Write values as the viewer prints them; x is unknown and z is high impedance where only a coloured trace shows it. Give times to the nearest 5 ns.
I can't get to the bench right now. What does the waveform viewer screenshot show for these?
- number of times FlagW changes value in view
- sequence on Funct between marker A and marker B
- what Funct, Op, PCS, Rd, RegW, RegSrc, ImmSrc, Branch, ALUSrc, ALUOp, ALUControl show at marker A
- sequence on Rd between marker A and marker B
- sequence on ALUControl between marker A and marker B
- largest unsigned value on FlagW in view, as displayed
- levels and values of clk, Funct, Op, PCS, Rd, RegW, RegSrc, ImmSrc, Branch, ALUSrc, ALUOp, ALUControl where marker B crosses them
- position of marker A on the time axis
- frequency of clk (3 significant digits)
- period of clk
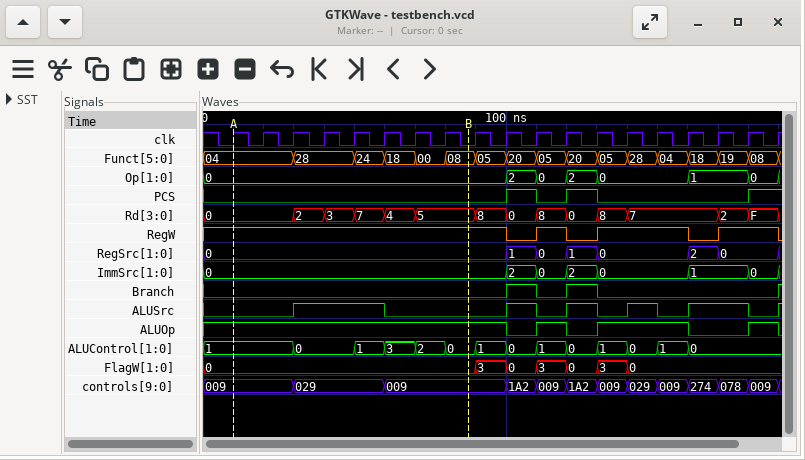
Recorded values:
6
04, 28, 24, 18, 00, 08
Funct=04, Op=0, PCS=0, Rd=0, RegW=1, RegSrc=0, ImmSrc=0, Branch=0, ALUSrc=0, ALUOp=1, ALUControl=1
0, 2, 3, 7, 4, 5
1, 0, 1, 3, 2, 0
3
clk=0, Funct=08, Op=0, PCS=0, Rd=5, RegW=1, RegSrc=0, ImmSrc=0, Branch=0, ALUSrc=0, ALUOp=1, ALUControl=0
10 ns
100 MHz
10 ns
